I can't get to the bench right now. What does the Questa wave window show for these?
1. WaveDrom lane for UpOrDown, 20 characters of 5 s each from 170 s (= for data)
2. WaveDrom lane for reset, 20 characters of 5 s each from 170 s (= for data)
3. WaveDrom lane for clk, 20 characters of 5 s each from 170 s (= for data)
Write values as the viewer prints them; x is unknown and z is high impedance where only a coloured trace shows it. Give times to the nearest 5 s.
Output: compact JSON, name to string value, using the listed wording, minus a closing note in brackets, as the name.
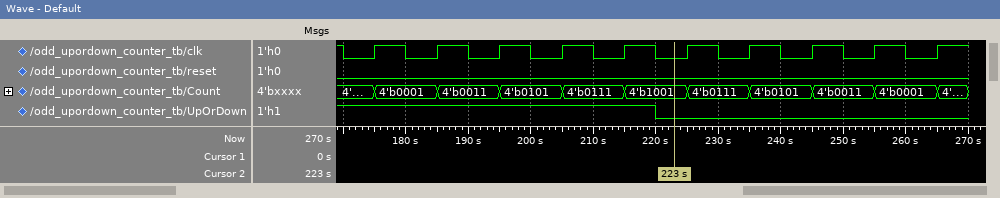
{"WaveDrom lane for UpOrDown, 20 characters of 5 s each from 170 s": "{name: 'UpOrDown', wave: '1.........0.........'}", "WaveDrom lane for reset, 20 characters of 5 s each from 170 s": "{name: 'reset', wave: '0...................'}", "WaveDrom lane for clk, 20 characters of 5 s each from 170 s": "{name: 'clk', wave: '01010101010101010101'}"}
